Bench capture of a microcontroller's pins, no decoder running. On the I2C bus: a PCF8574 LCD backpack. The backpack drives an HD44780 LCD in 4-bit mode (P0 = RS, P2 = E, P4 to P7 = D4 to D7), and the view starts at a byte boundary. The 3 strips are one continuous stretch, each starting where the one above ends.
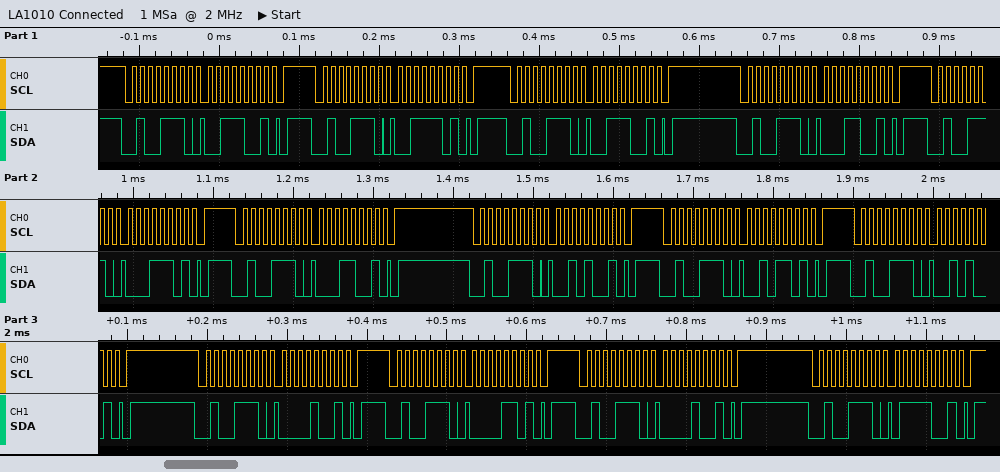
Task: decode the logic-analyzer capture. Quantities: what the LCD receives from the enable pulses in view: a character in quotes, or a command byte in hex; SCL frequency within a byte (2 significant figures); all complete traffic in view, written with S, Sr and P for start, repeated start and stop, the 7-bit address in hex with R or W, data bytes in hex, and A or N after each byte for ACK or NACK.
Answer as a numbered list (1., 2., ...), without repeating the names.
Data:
1. '1' ' '
2. 100 kHz
3. S 27W A 39 A P S 27W A 3D A P S 27W A 39 A P S 27W A 19 A P S 27W A 1D A P S 27W A 19 A P S 27W A 29 A P S 27W A 2D A P S 27W A 29 A P S 27W A 09 A P S 27W A 0D A P S 27W A 09 A P S 27W A 79 A P
